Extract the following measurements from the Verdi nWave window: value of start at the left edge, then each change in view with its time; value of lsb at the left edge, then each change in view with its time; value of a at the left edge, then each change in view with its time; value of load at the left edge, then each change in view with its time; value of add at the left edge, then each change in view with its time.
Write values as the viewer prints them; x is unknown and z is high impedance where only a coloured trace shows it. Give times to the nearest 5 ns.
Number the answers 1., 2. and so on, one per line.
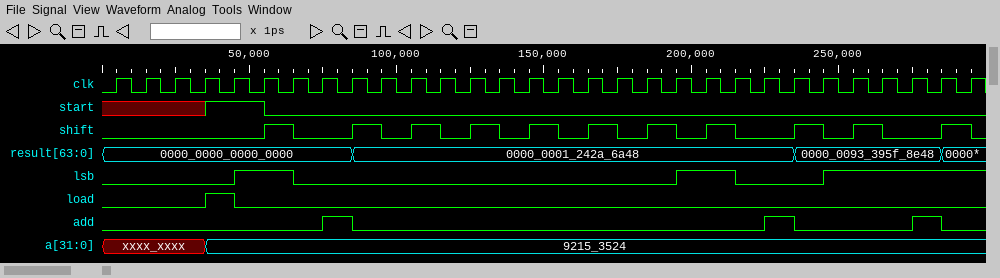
1. x, 1 at 35 ns, 0 at 55 ns
2. 0, 1 at 45 ns, 0 at 65 ns, 1 at 195 ns, 0 at 215 ns, 1 at 245 ns
3. xxxx_xxxx, 9215_3524 at 35 ns
4. 0, 1 at 35 ns, 0 at 45 ns
5. 0, 1 at 75 ns, 0 at 85 ns, 1 at 225 ns, 0 at 235 ns, 1 at 275 ns, 0 at 285 ns
